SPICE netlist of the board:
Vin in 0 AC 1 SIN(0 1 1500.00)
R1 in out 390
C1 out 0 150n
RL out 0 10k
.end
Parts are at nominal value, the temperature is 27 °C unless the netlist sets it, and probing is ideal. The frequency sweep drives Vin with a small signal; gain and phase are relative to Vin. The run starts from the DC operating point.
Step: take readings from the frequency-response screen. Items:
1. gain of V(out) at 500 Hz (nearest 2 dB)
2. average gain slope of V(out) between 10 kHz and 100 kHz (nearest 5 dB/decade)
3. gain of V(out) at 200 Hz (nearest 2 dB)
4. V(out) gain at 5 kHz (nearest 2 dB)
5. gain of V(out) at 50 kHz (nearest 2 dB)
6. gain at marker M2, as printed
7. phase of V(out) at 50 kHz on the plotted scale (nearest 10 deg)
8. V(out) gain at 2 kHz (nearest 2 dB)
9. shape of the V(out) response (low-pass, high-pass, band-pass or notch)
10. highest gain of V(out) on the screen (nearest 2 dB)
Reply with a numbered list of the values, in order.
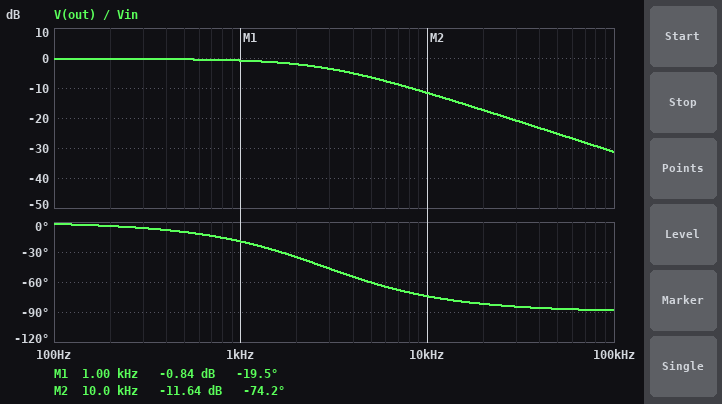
1. 0 dB
2. -20 dB/decade
3. 0 dB
4. -6 dB
5. -26 dB
6. -11.64 dB
7. -90 deg
8. -2 dB
9. low-pass
10. 0 dB
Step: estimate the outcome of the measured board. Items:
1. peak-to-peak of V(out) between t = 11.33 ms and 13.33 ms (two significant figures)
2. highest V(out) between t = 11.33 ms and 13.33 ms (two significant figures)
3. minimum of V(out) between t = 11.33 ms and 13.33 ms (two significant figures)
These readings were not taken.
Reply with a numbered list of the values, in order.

1. 1.7 V
2. 850 mV
3. -850 mV
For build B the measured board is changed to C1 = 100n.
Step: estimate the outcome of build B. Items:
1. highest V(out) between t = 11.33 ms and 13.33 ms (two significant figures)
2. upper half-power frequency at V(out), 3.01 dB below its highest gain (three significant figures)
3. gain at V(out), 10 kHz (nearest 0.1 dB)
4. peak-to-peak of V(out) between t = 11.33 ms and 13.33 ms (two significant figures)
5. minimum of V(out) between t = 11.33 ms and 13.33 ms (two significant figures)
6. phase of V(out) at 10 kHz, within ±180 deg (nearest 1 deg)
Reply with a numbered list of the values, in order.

1. 910 mV
2. 4.24 kHz
3. -8.5 dB
4. 1.8 V
5. -910 mV
6. -67 deg
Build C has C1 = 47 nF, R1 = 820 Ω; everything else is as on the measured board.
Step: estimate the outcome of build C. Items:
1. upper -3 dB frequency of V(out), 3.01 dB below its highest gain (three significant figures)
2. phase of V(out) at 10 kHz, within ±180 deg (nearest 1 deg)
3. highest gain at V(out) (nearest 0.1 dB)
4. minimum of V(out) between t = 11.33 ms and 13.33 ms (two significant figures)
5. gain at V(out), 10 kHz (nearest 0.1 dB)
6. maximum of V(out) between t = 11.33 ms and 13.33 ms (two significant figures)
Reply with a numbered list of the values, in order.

1. 4.47 kHz
2. -66 deg
3. -0.7 dB
4. -880 mV
5. -8.5 dB
6. 880 mV
